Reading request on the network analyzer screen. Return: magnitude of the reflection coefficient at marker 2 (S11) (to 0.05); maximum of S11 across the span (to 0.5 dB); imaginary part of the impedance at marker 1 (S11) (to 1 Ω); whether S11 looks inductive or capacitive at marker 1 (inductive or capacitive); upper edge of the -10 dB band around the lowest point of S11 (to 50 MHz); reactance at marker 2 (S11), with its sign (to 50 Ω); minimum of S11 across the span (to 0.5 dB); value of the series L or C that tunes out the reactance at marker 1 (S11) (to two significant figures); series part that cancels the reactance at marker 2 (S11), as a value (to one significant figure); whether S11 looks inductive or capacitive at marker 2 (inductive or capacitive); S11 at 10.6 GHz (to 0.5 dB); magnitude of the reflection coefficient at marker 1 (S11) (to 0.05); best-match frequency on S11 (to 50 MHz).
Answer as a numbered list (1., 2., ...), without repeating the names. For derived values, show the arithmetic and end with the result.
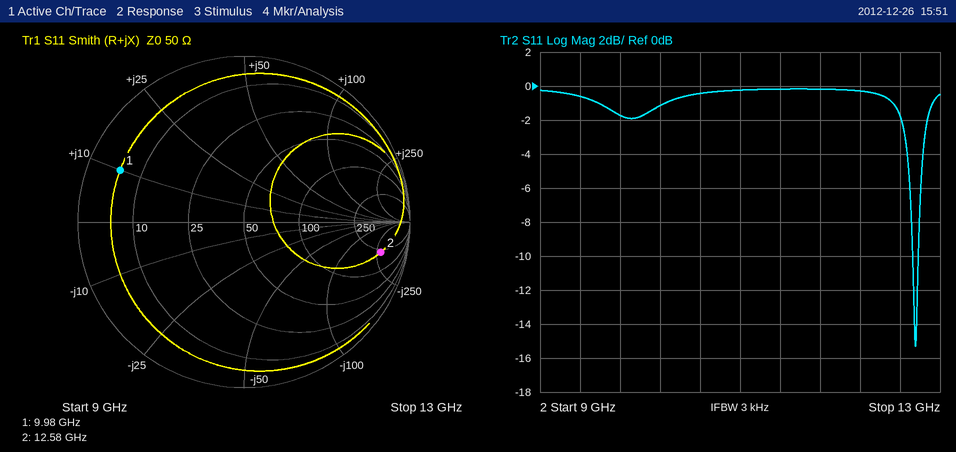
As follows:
1. 0.85
2. 0.0 dB
3. +10 Ω
4. inductive
5. 12.80 GHz
6. -300 Ω
7. -15.5 dB
8. C = 1/(2π × 9.98 GHz × 10 Ω) ≈ 1.6 pF
9. L = 300 Ω/(2π × 12.58 GHz) ≈ 4 nH
10. capacitive
11. -0.5 dB
12. 0.80
13. 12.75 GHz
